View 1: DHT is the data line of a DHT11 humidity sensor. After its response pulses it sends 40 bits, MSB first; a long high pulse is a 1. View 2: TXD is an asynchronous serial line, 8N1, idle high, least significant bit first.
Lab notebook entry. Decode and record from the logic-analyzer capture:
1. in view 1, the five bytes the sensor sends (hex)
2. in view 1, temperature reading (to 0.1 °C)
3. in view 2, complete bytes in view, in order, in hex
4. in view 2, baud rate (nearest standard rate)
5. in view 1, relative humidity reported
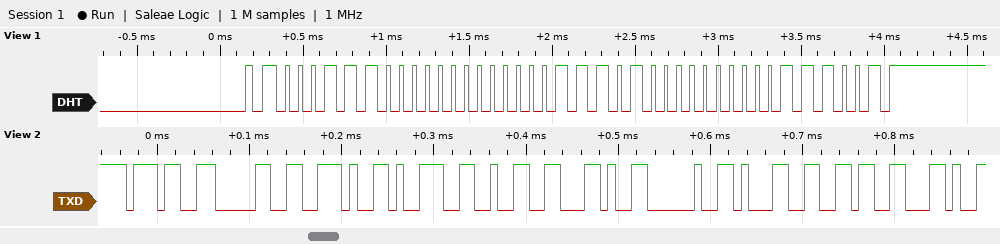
1C 00 1D 00 39
29.0 °C
0x37 0x30 0x2E 0x39 0x32 0x2C 0x20 0x31 0x36 0x2C
115200 baud
28 %
